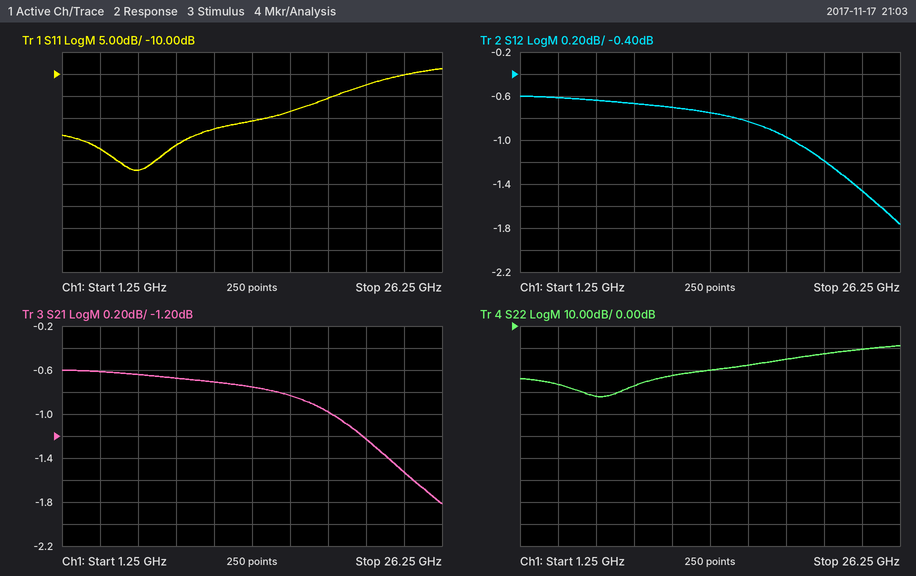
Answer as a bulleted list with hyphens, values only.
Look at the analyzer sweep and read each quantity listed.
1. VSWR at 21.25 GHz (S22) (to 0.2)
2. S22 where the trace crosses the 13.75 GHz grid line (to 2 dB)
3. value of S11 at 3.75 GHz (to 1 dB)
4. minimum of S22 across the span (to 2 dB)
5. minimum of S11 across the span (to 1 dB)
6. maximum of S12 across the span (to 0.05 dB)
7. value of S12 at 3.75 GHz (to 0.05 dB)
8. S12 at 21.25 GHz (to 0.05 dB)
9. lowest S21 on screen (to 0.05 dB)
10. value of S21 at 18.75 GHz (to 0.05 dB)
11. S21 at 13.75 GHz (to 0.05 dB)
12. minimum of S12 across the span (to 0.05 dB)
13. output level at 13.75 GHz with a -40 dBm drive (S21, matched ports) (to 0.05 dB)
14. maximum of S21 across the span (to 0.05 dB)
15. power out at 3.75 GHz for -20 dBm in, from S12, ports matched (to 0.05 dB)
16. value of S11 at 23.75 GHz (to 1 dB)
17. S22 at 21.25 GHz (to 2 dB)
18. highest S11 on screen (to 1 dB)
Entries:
- 1.6
- -20 dB
- -27 dB
- -32 dB
- -32 dB
- -0.60 dB
- -0.60 dB
- -1.20 dB
- -1.80 dB
- -1.00 dB
- -0.75 dB
- -1.75 dB
- -40.75 dBm
- -0.60 dB
- -20.60 dBm
- -10 dB
- -12 dB
- -9 dB
